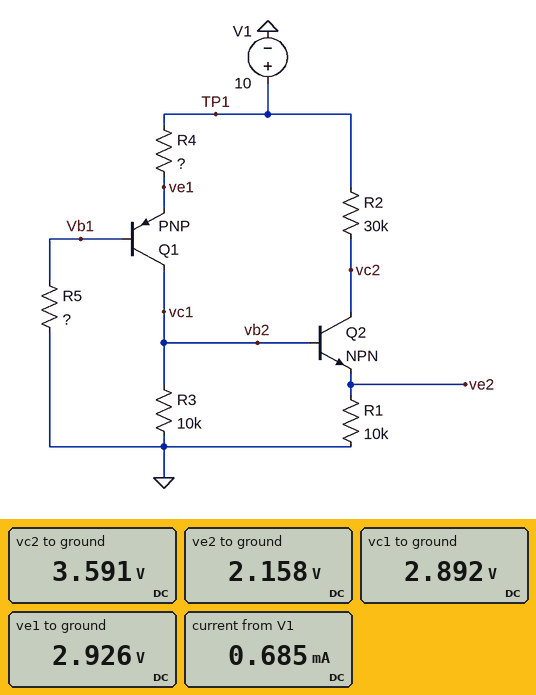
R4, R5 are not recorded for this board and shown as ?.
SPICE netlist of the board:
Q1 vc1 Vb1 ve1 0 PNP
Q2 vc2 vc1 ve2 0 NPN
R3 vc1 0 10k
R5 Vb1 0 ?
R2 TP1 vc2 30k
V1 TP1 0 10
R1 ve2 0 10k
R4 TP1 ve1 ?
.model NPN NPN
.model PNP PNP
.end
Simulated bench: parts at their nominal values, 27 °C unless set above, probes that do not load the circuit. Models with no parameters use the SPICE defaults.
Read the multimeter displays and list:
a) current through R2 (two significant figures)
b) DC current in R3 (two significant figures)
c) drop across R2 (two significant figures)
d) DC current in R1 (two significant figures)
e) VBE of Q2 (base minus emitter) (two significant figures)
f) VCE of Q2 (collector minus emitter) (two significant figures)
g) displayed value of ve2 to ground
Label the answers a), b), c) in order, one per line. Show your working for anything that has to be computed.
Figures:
a) (10 V - 3.591 V) / 30 kΩ = 210 µA
b) (2.892 V) / 10 kΩ = 290 µA
c) 10 V - 3.591 V = 6.4 V
d) (2.158 V) / 10 kΩ = 220 µA
e) 2.892 V - 2.158 V = 730 mV
f) 3.591 V - 2.158 V = 1.4 V
g) 2.158 V
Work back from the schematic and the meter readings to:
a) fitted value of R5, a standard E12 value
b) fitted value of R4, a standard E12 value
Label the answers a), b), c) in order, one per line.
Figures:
a) 12 kΩ
b) 15 kΩ
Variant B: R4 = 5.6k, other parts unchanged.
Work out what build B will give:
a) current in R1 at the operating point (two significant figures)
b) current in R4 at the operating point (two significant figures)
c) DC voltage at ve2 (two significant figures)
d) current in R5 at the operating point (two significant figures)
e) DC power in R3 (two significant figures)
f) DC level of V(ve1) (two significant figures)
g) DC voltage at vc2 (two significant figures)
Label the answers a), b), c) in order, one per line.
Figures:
a) 380 µA
b) 960 µA
c) 3.8 V
d) 320 µA
e) 2.1 mW
f) 4.6 V
g) 3.9 V
